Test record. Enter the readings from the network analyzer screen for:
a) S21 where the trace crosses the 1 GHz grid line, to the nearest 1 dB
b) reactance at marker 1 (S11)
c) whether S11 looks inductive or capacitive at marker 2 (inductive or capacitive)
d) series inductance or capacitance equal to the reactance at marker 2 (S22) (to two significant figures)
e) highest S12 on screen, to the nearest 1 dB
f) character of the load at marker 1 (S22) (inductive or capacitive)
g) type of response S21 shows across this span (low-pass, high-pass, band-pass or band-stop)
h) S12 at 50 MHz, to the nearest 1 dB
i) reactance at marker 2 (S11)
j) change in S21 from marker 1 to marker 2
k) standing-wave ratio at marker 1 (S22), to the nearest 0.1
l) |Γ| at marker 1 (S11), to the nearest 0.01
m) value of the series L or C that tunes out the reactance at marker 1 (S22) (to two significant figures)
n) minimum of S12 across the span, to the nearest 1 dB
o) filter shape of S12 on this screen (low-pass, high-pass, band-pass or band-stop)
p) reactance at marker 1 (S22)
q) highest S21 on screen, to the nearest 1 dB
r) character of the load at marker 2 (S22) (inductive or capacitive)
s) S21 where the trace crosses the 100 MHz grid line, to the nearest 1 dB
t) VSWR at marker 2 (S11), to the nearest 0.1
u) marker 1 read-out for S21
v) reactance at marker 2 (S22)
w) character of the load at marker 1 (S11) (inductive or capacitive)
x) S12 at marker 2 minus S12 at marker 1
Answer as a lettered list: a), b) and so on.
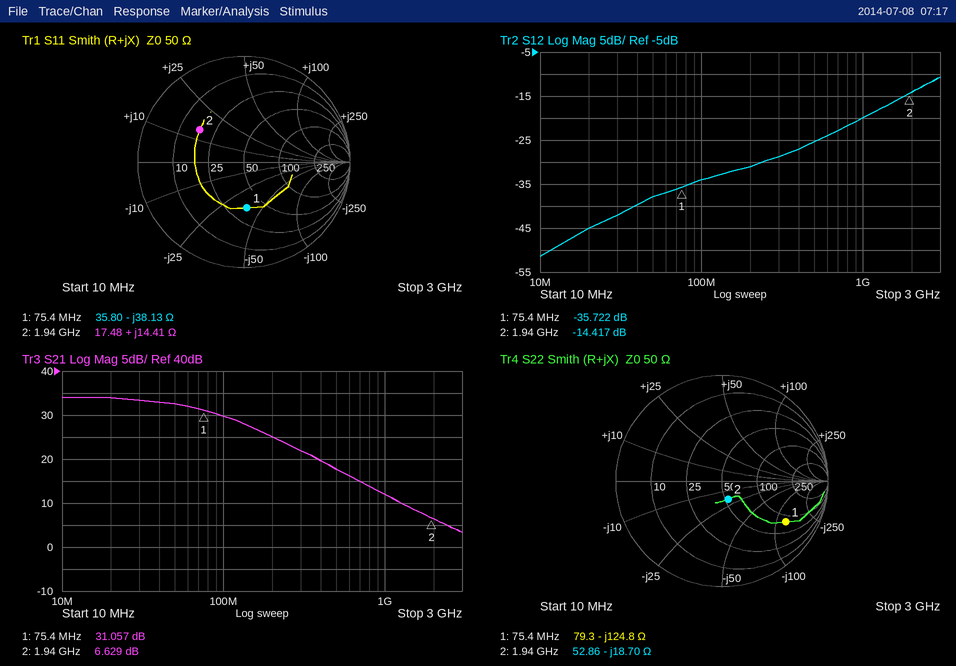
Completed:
a) 12 dB
b) -38.13 Ω
c) inductive
d) 4.4 pF
e) -11 dB
f) capacitive
g) low-pass
h) -38 dB
i) +14.41 Ω
j) -24.428 dB
k) 6.0
l) 0.43
m) 260 nH
n) -51 dB
o) high-pass
p) -124.8 Ω
q) 34 dB
r) capacitive
s) 30 dB
t) 3.1
u) 31.057 dB
v) -18.70 Ω
w) capacitive
x) 21.305 dB
